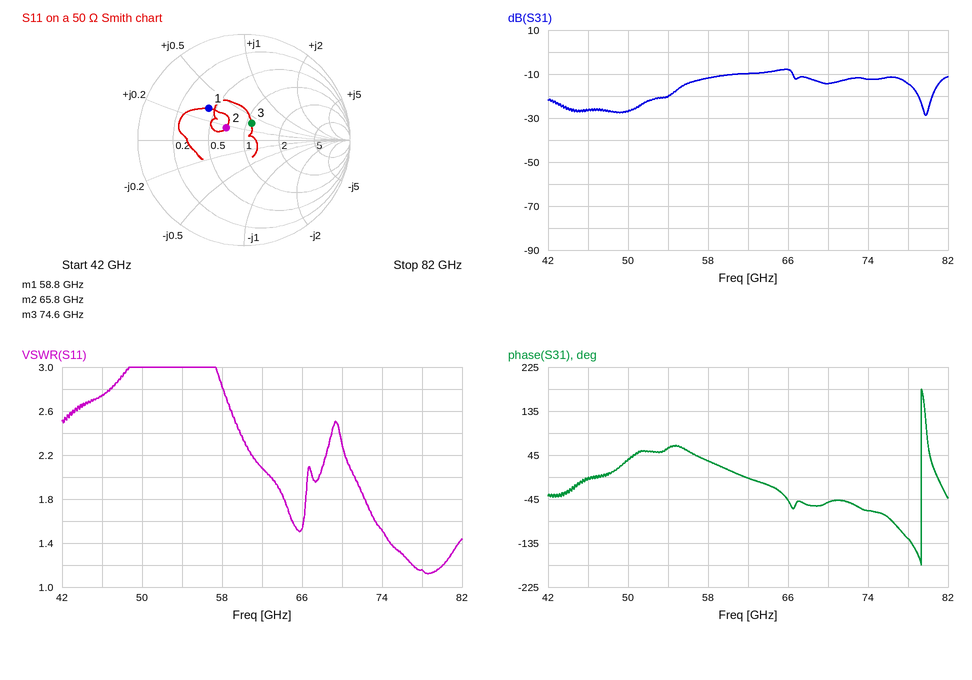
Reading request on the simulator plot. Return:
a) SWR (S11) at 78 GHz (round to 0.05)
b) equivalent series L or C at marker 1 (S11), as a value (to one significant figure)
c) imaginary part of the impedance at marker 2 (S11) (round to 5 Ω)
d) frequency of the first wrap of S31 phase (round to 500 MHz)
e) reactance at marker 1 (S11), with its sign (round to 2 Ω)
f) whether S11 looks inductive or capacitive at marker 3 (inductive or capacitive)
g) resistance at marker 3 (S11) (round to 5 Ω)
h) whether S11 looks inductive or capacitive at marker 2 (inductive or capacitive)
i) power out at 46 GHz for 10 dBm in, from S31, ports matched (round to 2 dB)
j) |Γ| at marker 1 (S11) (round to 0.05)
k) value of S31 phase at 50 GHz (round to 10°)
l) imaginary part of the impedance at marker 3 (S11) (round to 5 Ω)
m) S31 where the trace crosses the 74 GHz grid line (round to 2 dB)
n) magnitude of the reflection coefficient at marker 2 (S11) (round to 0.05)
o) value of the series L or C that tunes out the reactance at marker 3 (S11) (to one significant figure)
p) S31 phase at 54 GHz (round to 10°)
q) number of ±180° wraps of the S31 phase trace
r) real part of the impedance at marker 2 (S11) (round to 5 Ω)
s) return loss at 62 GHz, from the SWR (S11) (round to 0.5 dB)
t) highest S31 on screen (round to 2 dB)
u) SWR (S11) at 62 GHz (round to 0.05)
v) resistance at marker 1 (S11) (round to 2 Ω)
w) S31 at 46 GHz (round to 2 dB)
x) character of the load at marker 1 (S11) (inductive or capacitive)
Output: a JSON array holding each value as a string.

["1.15", "40 pH", "+10 Ω", "79.5 GHz", "+16 Ω", "inductive", "55 Ω", "inductive", "-16 dBm", "0.45", "40°", "+20 Ω", "-12 dB", "0.20", "100 fF", "60°", "1", "35 Ω", "9.0 dB", "-8 dB", "2.10", "22 Ω", "-26 dB", "inductive"]
